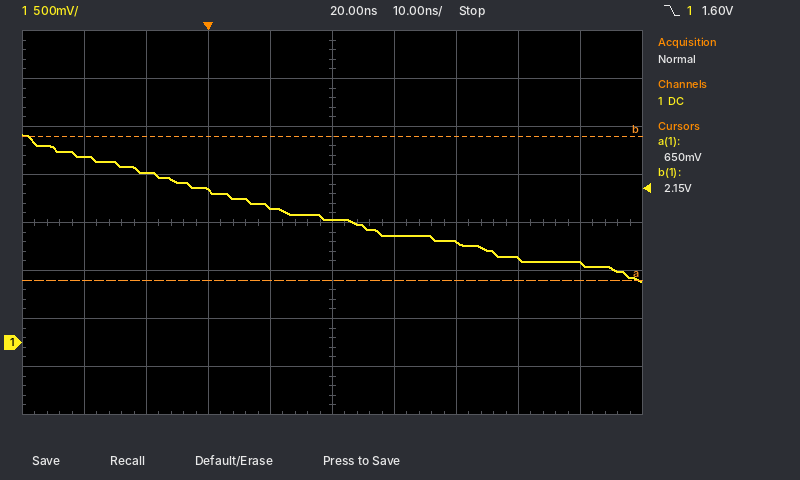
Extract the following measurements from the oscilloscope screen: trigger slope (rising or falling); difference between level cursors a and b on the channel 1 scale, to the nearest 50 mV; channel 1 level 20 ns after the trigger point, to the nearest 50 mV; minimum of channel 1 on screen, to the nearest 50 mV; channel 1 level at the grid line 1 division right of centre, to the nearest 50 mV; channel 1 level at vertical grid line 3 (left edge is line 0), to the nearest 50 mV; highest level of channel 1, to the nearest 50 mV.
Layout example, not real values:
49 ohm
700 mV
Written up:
falling
1.50 V
1.30 V
650 mV
1.10 V
1.60 V
2.15 V
